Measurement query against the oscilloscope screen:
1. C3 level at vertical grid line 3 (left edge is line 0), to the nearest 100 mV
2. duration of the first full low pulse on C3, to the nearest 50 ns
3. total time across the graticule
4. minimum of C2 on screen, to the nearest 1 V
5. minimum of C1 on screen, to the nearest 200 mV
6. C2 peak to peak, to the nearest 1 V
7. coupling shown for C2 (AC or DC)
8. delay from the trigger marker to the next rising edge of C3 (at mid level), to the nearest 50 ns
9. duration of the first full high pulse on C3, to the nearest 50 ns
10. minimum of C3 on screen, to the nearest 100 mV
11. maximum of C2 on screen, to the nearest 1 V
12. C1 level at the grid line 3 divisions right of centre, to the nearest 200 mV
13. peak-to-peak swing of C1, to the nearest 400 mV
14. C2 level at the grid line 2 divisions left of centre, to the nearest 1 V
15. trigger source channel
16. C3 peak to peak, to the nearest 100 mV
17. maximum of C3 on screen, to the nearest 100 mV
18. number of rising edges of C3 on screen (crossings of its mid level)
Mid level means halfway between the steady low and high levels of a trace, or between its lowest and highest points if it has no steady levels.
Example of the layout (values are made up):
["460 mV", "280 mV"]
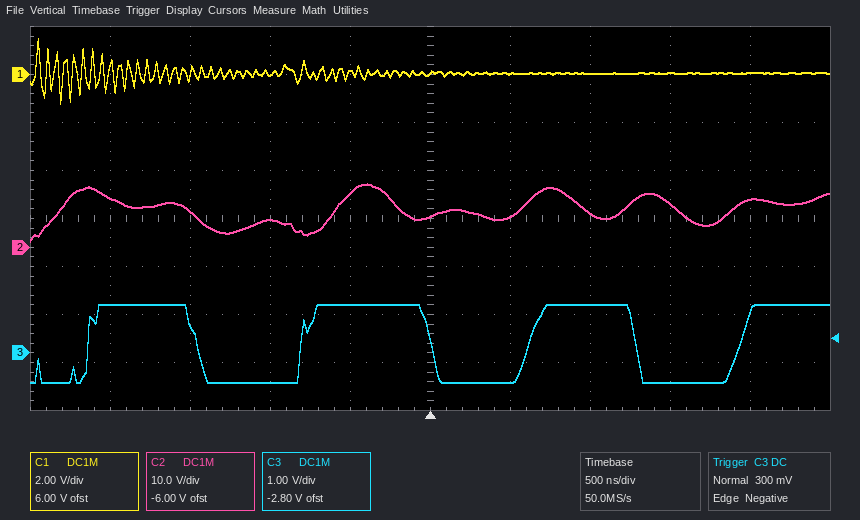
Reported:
["-600 mV", "650 ns", "5 µs", "1 V", "-1.2 V", "12 V", "DC", "600 ns", "700 ns", "-600 mV", "13 V", "0.0 V", "2.8 V", "6 V", "C3", "1.6 V", "1.0 V", "4"]
